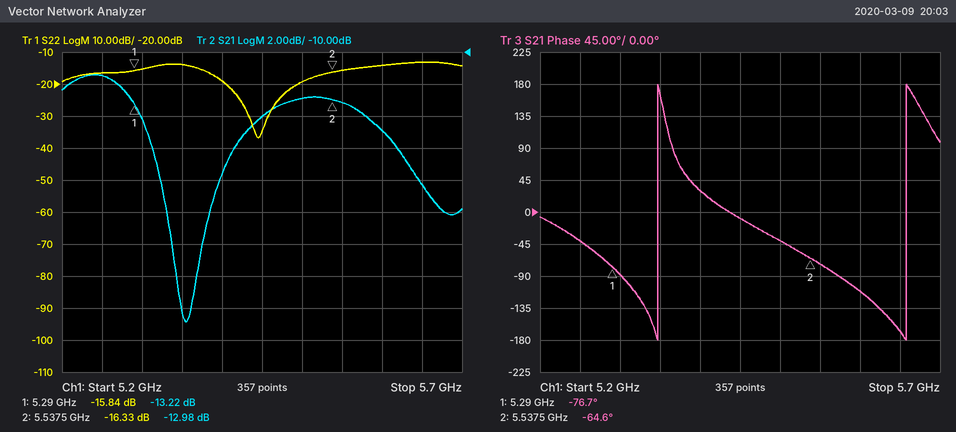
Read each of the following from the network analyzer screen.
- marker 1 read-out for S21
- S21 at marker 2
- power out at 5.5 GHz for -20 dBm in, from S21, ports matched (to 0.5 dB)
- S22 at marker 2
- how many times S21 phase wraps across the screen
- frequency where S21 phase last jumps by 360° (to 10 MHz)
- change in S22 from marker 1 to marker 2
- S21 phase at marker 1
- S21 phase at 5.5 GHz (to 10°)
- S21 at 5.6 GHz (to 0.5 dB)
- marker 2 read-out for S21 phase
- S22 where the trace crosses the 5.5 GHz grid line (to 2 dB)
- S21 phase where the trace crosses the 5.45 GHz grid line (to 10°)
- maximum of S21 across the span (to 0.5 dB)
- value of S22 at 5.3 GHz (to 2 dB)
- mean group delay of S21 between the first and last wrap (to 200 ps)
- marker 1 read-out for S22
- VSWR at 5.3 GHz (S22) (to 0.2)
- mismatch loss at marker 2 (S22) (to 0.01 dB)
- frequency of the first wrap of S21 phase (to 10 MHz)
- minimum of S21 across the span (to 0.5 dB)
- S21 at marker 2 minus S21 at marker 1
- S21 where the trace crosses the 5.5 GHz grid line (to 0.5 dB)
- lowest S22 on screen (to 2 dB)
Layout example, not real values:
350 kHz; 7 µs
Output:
-13.22 dB; -12.98 dB; -33.0 dBm; -16.33 dB; 2; 5.66 GHz; -0.49 dB; -76.7°; -40°; -15.0 dB; -64.6°; -20 dB; -10°; -11.5 dB; -16 dB; 3.2 ns; -15.84 dB; 1.4; 0.10 dB; 5.35 GHz; -27.0 dB; 0.24 dB; -13.0 dB; -36 dB
